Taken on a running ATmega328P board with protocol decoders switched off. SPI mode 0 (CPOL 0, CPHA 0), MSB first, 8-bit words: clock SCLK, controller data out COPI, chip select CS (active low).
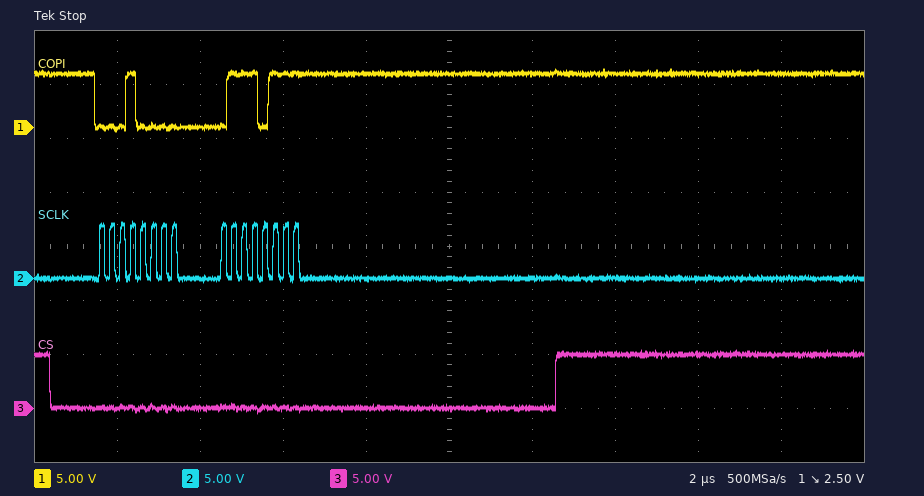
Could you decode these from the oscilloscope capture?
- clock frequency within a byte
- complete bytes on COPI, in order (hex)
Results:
4 MHz
10 77
